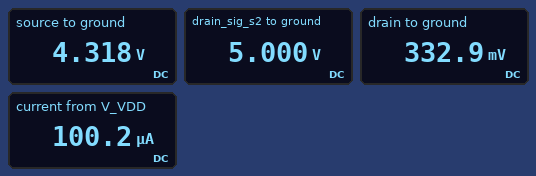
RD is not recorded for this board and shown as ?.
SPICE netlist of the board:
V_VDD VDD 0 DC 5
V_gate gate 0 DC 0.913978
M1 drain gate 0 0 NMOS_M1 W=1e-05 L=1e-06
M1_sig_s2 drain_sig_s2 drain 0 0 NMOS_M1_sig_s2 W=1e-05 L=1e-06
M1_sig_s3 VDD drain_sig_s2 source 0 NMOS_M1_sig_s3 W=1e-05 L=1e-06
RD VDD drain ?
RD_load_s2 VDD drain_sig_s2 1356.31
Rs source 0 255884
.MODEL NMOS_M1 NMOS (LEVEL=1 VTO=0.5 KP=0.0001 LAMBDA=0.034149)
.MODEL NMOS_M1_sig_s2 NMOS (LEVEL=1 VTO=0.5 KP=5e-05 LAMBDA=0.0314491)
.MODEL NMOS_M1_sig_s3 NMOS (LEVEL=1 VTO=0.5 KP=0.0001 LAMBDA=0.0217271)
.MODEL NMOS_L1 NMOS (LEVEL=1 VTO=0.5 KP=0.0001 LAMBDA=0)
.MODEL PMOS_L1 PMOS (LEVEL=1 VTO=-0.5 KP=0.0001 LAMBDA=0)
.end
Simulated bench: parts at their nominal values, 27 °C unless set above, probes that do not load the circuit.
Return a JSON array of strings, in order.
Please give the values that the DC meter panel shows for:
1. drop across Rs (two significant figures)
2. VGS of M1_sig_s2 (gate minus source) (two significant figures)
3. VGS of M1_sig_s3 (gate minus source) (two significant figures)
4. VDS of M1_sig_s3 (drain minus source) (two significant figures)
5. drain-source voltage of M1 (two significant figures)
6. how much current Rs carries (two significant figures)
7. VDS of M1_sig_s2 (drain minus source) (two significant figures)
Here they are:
["4.3 V", "330 mV", "680 mV", "680 mV", "330 mV", "17 µA", "5.0 V"]
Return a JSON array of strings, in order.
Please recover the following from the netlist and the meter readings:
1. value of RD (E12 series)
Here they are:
["56 kΩ"]
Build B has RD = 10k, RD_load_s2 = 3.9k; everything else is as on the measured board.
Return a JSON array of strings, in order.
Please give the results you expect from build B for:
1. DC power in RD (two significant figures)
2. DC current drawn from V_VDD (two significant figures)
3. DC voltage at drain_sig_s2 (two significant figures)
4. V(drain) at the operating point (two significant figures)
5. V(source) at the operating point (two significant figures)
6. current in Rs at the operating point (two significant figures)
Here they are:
["95 µW", "1.2 mA", "680 mV", "4.0 V", "150 mV", "580 nA"]
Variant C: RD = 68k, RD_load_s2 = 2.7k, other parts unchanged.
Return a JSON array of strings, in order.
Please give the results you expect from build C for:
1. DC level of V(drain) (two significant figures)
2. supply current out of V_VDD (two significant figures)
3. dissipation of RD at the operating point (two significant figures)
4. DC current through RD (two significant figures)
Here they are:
["230 mV", "87 µA", "330 µW", "70 µA"]
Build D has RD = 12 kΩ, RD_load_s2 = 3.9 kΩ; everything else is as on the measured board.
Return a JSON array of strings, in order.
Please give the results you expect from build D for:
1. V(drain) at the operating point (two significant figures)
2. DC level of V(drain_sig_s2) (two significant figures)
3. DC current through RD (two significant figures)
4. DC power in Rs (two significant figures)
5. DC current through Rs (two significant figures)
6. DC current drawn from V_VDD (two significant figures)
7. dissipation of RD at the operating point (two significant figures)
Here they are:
["3.8 V", "720 mV", "97 µA", "130 nW", "720 nA", "1.2 mA", "110 µW"]
